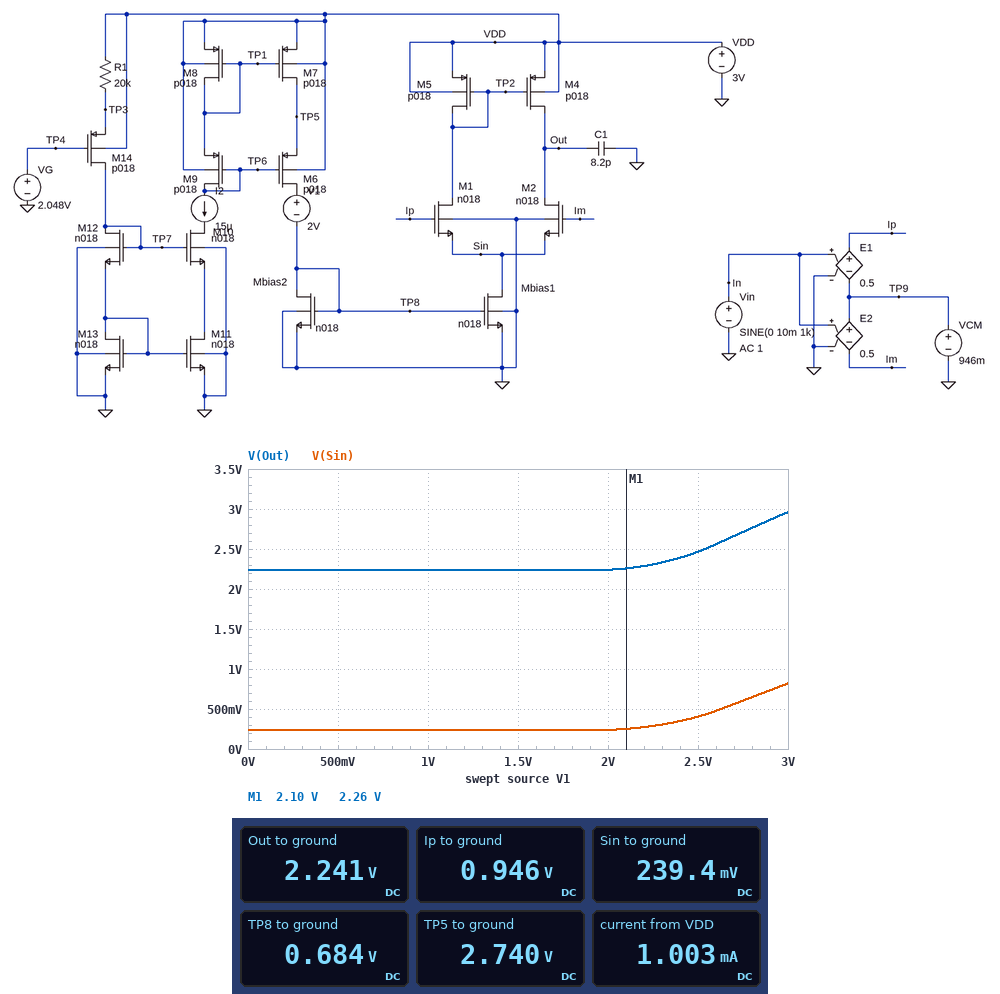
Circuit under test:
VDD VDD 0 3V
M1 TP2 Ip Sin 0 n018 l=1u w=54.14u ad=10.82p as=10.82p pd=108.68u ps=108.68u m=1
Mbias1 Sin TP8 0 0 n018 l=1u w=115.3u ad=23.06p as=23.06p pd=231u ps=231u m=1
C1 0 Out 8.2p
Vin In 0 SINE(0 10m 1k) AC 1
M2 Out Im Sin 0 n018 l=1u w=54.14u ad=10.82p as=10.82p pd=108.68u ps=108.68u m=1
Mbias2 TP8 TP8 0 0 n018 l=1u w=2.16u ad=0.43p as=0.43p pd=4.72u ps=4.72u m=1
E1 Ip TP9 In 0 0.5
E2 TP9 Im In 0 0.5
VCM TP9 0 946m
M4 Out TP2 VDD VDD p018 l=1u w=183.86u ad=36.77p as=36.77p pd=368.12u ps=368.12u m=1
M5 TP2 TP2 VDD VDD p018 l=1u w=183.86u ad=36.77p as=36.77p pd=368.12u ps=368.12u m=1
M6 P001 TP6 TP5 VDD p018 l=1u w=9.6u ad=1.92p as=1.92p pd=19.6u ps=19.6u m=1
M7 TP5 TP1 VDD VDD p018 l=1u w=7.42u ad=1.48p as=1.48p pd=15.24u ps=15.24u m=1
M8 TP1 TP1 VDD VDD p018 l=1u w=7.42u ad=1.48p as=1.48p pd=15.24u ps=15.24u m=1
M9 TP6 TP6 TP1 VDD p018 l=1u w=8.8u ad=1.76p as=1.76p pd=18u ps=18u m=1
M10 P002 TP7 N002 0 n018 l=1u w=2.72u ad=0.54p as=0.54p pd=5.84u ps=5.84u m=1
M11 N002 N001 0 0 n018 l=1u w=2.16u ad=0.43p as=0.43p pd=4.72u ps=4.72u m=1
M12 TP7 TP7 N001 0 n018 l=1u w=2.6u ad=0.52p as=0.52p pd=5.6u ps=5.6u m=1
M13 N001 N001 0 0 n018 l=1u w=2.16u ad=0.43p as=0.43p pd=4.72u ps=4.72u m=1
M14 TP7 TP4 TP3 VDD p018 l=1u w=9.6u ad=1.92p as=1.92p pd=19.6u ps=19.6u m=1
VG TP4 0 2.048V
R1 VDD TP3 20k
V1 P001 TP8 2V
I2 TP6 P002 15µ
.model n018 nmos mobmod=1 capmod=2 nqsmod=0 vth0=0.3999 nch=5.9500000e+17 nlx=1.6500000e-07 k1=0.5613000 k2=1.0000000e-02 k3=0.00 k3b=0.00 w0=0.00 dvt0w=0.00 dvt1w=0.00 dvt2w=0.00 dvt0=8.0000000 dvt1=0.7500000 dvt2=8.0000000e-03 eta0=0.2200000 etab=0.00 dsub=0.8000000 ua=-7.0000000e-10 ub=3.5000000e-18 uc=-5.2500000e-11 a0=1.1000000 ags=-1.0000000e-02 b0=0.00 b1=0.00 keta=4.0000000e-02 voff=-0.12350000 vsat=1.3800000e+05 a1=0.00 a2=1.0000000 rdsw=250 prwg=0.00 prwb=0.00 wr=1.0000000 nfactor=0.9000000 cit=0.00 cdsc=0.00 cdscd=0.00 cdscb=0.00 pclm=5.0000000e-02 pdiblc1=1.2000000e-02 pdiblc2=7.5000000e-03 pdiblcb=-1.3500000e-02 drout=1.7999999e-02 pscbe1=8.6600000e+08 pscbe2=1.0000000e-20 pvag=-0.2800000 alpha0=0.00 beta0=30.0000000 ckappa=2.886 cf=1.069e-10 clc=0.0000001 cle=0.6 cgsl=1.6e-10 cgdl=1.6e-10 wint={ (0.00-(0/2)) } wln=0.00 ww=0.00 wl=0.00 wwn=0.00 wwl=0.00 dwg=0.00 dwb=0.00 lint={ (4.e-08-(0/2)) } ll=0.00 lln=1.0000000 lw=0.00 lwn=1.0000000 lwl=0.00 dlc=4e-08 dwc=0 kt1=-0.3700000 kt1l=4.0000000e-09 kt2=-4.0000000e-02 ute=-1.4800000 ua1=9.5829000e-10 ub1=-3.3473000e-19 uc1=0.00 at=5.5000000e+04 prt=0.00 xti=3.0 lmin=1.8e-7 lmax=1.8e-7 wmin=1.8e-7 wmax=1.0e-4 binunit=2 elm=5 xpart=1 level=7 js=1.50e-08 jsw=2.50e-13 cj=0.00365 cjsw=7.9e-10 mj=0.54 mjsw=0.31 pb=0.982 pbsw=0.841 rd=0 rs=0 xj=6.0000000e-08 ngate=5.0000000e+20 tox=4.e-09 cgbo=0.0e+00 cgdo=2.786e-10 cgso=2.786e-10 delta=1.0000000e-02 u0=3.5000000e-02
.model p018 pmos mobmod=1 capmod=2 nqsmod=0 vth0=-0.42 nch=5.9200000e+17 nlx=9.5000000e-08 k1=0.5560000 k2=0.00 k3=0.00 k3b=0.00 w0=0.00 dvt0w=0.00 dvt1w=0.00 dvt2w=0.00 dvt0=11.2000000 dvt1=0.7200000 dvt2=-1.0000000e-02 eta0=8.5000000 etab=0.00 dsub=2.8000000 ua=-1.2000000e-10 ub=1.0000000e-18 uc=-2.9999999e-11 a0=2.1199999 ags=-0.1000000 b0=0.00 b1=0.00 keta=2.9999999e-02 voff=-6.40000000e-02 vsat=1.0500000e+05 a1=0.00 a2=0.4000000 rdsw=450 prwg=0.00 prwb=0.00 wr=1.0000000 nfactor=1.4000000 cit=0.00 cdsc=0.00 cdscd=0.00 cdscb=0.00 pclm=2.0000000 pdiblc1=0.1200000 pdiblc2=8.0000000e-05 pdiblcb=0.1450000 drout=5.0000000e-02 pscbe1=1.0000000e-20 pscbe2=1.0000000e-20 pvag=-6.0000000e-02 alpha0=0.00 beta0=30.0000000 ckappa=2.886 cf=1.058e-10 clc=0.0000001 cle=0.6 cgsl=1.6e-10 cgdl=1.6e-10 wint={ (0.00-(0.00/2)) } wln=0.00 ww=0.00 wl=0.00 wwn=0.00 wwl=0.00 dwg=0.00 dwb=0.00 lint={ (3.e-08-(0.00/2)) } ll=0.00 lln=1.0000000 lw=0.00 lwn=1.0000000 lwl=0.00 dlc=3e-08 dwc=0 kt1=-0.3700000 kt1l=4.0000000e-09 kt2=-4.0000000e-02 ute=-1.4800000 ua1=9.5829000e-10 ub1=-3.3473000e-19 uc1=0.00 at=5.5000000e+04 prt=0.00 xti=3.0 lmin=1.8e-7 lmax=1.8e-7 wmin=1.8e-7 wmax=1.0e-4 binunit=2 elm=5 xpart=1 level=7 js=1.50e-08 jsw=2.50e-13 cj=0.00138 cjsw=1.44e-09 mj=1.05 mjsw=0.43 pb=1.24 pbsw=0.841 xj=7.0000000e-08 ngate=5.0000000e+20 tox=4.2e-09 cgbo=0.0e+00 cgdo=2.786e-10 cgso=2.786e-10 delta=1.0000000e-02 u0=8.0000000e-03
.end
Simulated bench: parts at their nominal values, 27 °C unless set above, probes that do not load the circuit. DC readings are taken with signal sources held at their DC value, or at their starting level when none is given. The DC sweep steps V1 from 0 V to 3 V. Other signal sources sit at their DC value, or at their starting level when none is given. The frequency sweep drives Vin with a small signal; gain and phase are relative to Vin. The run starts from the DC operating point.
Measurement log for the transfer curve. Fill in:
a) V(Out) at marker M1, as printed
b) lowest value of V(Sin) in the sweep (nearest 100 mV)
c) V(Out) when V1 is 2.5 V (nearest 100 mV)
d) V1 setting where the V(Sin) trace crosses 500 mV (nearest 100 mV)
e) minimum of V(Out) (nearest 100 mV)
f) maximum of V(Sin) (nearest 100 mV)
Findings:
2.26 V
200 mV
2.5 V
2.6 V
2.2 V
800 mV
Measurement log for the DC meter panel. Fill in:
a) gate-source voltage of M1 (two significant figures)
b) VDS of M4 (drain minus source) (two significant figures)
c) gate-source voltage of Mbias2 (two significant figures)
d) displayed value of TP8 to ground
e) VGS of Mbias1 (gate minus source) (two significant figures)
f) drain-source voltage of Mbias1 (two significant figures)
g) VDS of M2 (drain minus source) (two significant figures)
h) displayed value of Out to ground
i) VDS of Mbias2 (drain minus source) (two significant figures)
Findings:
710 mV
-760 mV
680 mV
0.684 V
680 mV
240 mV
2.0 V
2.241 V
680 mV
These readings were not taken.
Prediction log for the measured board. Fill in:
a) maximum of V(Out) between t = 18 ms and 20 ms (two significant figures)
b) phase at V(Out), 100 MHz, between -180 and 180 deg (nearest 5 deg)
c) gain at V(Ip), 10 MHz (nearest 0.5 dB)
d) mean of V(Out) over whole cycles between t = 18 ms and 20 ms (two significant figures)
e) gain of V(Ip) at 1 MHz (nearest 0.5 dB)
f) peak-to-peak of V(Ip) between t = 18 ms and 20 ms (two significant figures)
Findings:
2.5 V
-110 deg
-6.0 dB
2.2 V
-6.0 dB
10 mV
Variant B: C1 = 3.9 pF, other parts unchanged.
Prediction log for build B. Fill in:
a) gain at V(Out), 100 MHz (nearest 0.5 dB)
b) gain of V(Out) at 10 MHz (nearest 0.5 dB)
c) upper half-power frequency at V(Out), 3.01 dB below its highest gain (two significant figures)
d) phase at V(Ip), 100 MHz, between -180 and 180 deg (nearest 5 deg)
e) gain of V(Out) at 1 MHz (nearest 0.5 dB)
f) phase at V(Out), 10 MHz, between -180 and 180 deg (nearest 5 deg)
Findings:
-2.5 dB
18.5 dB
2.6 MHz
0 deg
30.0 dB
-80 deg
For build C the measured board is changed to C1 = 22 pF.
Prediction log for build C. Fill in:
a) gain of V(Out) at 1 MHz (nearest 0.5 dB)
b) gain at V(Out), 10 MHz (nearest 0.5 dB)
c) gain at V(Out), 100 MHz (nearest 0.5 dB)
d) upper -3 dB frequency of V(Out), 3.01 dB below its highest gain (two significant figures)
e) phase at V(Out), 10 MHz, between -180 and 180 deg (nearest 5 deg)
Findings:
24.0 dB
5.0 dB
-16.5 dB
520 kHz
-90 deg
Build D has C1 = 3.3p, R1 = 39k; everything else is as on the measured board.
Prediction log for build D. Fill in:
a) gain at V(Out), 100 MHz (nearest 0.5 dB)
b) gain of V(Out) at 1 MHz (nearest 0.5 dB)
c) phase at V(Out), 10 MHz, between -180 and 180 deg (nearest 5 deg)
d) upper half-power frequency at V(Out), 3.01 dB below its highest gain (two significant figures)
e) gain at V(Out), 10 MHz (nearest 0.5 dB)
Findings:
-1.0 dB
30.5 dB
-75 deg
3.0 MHz
20.0 dB
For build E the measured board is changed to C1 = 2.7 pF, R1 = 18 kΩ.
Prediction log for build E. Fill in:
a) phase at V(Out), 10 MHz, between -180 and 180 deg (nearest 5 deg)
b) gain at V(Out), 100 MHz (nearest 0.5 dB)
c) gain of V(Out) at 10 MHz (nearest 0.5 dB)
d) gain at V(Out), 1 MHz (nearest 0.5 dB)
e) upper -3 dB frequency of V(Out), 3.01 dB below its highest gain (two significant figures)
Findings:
-75 deg
0.5 dB
21.0 dB
30.5 dB
3.5 MHz
